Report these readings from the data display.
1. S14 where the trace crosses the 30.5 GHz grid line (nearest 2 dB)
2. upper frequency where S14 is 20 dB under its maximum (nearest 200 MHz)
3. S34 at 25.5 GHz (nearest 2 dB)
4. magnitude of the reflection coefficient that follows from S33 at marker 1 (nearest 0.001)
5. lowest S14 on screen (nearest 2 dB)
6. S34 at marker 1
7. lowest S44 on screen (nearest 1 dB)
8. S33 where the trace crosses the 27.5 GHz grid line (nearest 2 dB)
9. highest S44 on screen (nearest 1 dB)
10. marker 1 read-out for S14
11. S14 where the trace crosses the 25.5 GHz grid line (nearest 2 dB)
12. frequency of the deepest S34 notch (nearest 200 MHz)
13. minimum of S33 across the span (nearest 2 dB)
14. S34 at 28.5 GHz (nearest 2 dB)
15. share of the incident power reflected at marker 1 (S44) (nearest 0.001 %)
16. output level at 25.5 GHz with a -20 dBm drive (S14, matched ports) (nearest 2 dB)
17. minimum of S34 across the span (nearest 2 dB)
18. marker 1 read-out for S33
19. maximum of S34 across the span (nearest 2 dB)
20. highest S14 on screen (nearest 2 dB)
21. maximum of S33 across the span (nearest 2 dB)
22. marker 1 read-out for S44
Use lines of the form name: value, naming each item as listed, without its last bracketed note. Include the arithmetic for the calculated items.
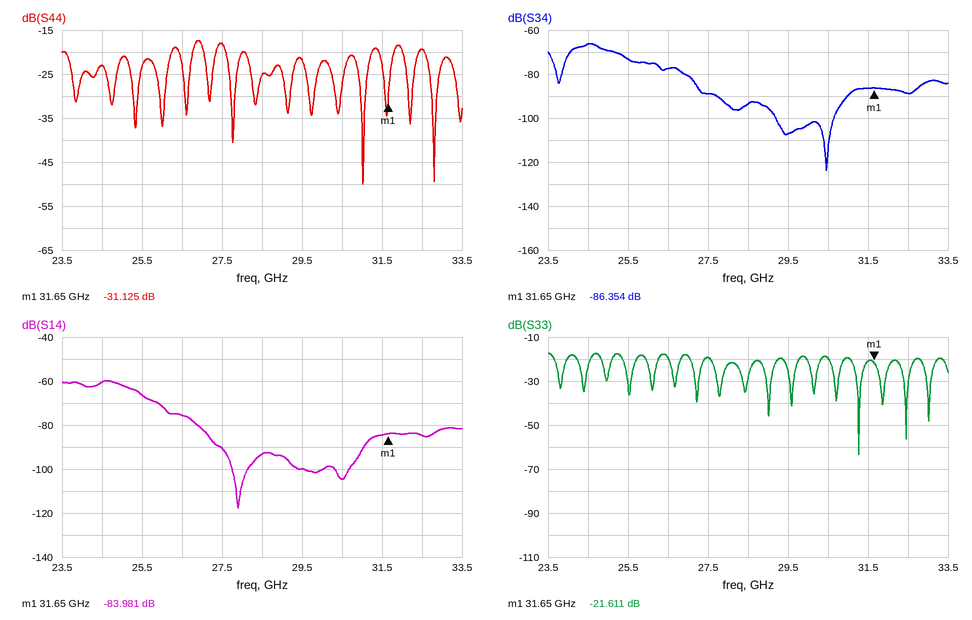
S14 where the trace crosses the 30.5 GHz grid line: -104 dB
upper frequency where S14 is 20 dB under its maximum: 26.8 GHz
S34 at 25.5 GHz: -74 dB
magnitude of the reflection coefficient that follows from S33 at marker 1: 10^(-21.611/20) ≈ 0.083
lowest S14 on screen: -118 dB
S34 at marker 1: -86.354 dB
lowest S44 on screen: -50 dB
S33 where the trace crosses the 27.5 GHz grid line: -20 dB
highest S44 on screen: -17 dB
marker 1 read-out for S14: -83.981 dB
S14 where the trace crosses the 25.5 GHz grid line: -66 dB
frequency of the deepest S34 notch: 30.4 GHz
minimum of S33 across the span: -64 dB
S34 at 28.5 GHz: -94 dB
share of the incident power reflected at marker 1 (S44): 10^(-31.125/10) ≈ 0.077 %
output level at 25.5 GHz with a -20 dBm drive (S14, matched ports): -20 dBm + (-66 dB) = -86 dBm
minimum of S34 across the span: -124 dB
marker 1 read-out for S33: -21.611 dB
maximum of S34 across the span: -66 dB
highest S14 on screen: -60 dB
maximum of S33 across the span: -18 dB
marker 1 read-out for S44: -31.125 dB
